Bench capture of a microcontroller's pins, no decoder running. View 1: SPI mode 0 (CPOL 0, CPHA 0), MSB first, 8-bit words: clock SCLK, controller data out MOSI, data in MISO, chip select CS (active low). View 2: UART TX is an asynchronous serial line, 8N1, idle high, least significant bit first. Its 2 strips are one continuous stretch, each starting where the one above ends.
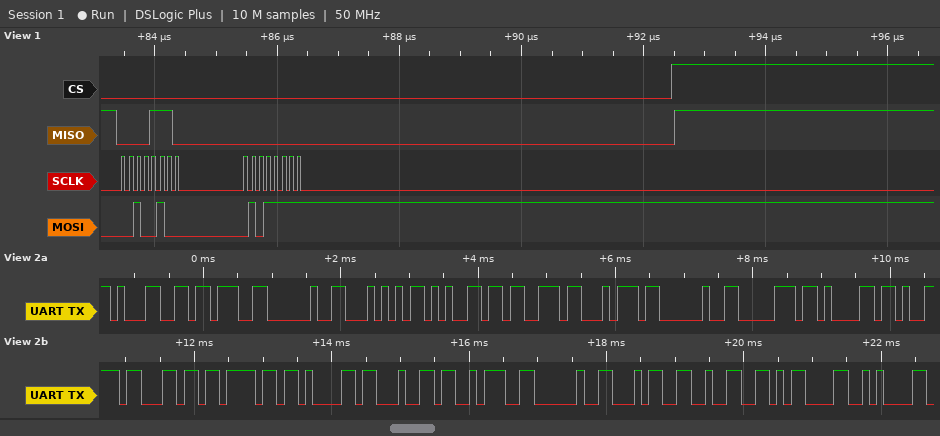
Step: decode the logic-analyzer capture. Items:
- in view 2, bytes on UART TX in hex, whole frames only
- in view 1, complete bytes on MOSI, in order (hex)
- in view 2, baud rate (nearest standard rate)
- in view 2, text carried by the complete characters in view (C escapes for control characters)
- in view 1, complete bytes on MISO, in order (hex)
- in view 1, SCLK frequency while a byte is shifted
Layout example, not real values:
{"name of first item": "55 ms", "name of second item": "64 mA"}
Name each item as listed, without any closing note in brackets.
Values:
{"in view 2, bytes on UART TX in hex, whole frames only": "0x31 0x3B 0x20 0x54 0x65 0x73 0x74 0x20 0x70 0x61 0x79 0x6C 0x6F 0x61 0x64 0x3A 0x20 0x34 0x32 0x0D 0x0A", "in view 1, complete bytes on MOSI, in order": "24 5F", "in view 2, baud rate": "9600 baud", "in view 2, text carried by the complete characters in view": "\"1; Test payload: 42\\r\\n\"", "in view 1, complete bytes on MISO, in order": "0E 00", "in view 1, SCLK frequency while a byte is shifted": "8 MHz"}
